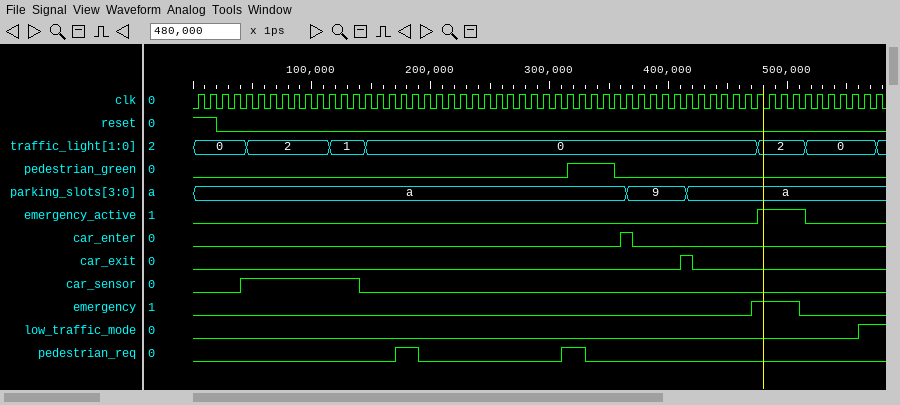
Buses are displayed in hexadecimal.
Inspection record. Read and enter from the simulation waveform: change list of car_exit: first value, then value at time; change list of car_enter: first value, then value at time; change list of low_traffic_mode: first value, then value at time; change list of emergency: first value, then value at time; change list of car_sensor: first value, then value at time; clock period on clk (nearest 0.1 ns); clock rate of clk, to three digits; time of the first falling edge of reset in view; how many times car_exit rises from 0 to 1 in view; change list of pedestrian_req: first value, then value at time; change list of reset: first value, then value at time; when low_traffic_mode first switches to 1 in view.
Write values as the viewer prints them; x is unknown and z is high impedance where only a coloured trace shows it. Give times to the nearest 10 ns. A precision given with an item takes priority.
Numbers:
0, 1 at 410 ns, 0 at 420 ns
0, 1 at 360 ns, 0 at 370 ns
0, 1 at 560 ns
0, 1 at 470 ns, 0 at 510 ns
0, 1 at 40 ns, 0 at 140 ns
10 ns
100 MHz
20 ns
1
0, 1 at 170 ns, 0 at 190 ns, 1 at 310 ns, 0 at 330 ns
1, 0 at 20 ns
560 ns
